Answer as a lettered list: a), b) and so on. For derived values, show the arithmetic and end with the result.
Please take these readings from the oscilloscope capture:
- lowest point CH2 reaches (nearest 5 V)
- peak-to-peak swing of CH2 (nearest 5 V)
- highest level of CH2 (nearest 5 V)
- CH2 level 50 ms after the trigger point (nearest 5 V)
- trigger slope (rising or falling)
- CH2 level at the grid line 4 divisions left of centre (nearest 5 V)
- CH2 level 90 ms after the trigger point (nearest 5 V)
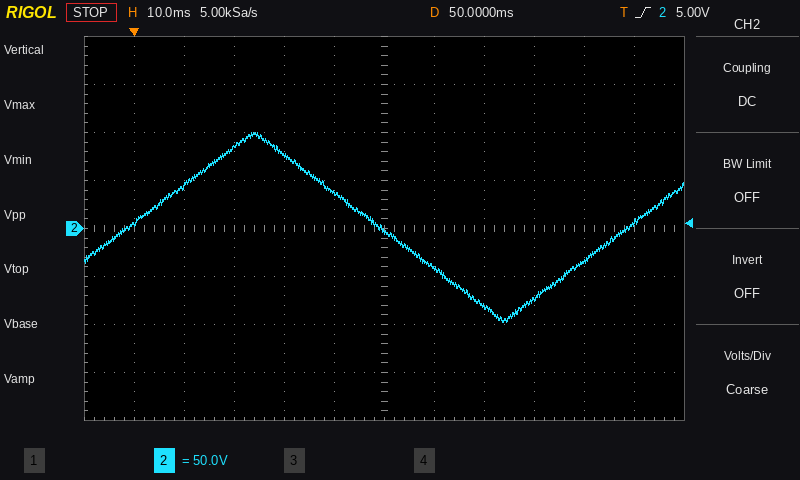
a) -100 V
b) 100 V − (-100 V) = 200 V
c) 100 V
d) 0 V
e) rising
f) 45 V
g) -35 V
